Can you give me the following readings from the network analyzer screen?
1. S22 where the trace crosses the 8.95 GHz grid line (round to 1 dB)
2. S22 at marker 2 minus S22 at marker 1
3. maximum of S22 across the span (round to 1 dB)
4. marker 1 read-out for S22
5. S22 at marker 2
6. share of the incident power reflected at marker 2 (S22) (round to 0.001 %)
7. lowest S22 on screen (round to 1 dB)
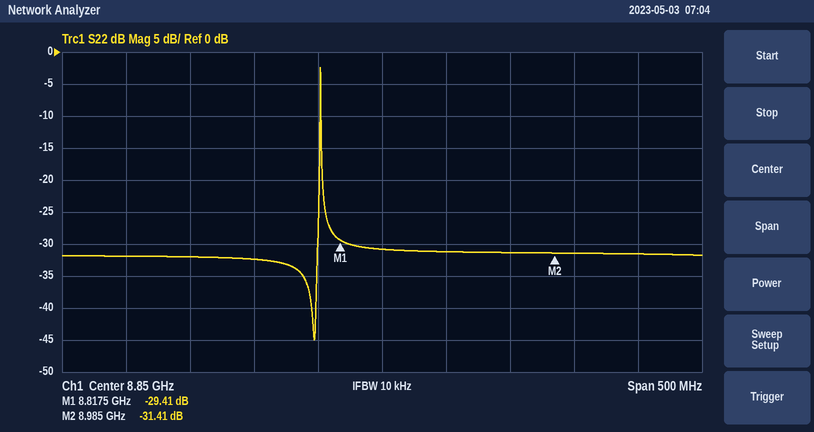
-31 dB
-2.00 dB
-2 dB
-29.41 dB
-31.41 dB
0.072 %
-45 dB
